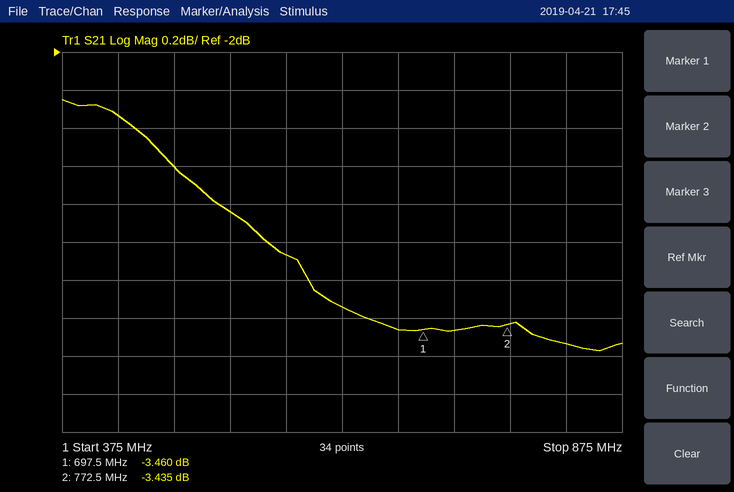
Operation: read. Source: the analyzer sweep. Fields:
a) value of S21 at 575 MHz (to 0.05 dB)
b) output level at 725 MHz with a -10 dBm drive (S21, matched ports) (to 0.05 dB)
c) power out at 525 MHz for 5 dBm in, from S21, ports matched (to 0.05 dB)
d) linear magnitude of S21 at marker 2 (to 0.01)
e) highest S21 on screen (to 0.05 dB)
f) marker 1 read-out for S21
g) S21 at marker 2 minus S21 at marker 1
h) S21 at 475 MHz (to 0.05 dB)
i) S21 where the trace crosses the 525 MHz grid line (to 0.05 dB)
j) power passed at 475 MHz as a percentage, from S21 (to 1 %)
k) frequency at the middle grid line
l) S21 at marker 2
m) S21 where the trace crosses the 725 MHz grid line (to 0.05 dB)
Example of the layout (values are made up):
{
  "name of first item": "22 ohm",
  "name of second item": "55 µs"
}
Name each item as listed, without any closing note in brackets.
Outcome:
{
  "value of S21 at 575 MHz": "-3.05 dB",
  "output level at 725 MHz with a -10 dBm drive (S21, matched ports)": "-13.45 dBm",
  "power out at 525 MHz for 5 dBm in, from S21, ports matched": "2.15 dBm",
  "linear magnitude of S21 at marker 2": "0.67",
  "highest S21 on screen": "-2.25 dB",
  "marker 1 read-out for S21": "-3.460 dB",
  "S21 at marker 2 minus S21 at marker 1": "0.025 dB",
  "S21 at 475 MHz": "-2.60 dB",
  "S21 where the trace crosses the 525 MHz grid line": "-2.85 dB",
  "power passed at 475 MHz as a percentage, from S21": "55 %",
  "frequency at the middle grid line": "625 MHz",
  "S21 at marker 2": "-3.435 dB",
  "S21 where the trace crosses the 725 MHz grid line": "-3.45 dB"
}
